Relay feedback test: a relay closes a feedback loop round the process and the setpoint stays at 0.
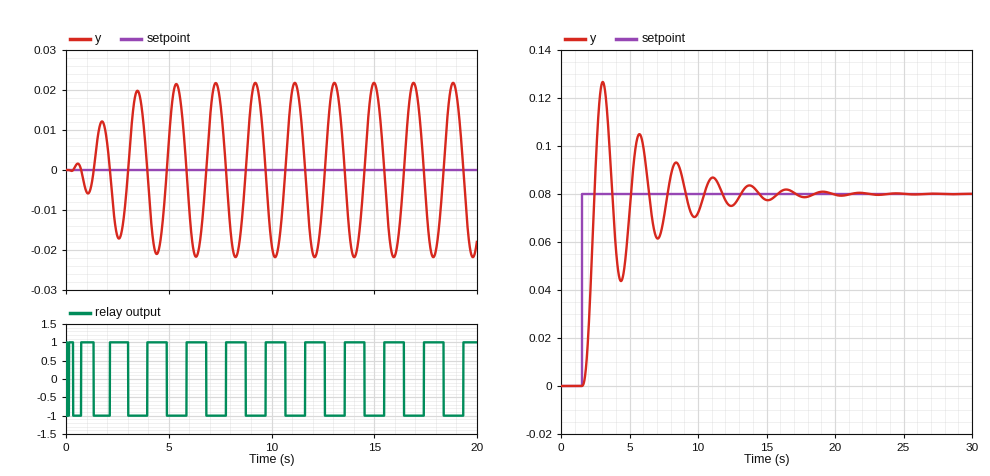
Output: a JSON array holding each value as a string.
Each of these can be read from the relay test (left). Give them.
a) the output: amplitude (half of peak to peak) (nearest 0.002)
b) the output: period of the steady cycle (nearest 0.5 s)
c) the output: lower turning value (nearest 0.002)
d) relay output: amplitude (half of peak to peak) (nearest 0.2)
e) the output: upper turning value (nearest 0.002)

["0.022", "2.0 s", "-0.022", "1.0", "0.022"]
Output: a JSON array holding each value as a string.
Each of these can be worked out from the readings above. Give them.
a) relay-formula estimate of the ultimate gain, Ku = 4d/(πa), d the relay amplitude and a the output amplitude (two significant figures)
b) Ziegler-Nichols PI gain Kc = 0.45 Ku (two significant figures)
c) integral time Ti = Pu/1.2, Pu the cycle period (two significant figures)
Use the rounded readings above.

["58", "26", "1.7 s"]
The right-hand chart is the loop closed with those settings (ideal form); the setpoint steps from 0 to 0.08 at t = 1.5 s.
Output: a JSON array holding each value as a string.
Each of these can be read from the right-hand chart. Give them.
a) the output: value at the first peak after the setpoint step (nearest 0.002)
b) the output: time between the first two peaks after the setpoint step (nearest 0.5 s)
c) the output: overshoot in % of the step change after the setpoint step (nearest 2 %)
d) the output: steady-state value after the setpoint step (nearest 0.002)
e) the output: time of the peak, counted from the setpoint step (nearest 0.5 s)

["0.126", "2.5 s", "58 %", "0.080", "1.5 s"]
